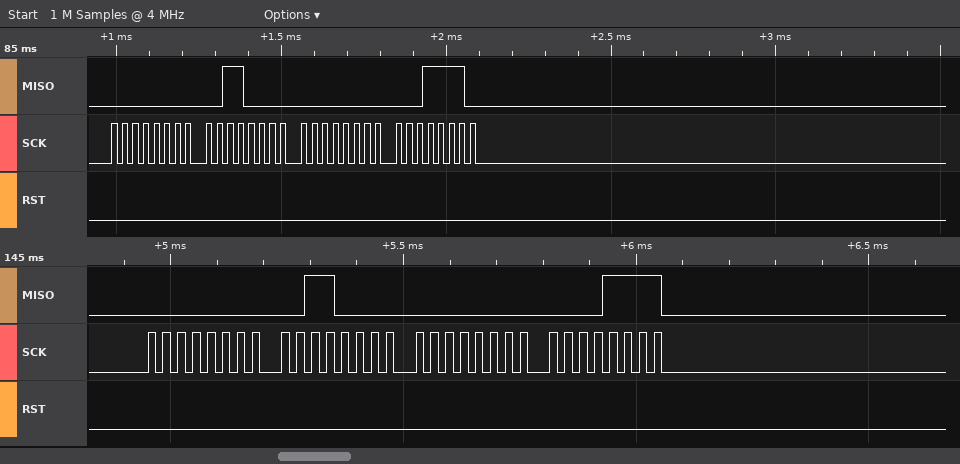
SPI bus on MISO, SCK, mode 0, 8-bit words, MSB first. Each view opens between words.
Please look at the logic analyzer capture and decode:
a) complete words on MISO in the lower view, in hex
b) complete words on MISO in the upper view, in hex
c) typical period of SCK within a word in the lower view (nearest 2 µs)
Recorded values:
00, 30, 00, 0F
00, 30, 00, 1E
32 µs
